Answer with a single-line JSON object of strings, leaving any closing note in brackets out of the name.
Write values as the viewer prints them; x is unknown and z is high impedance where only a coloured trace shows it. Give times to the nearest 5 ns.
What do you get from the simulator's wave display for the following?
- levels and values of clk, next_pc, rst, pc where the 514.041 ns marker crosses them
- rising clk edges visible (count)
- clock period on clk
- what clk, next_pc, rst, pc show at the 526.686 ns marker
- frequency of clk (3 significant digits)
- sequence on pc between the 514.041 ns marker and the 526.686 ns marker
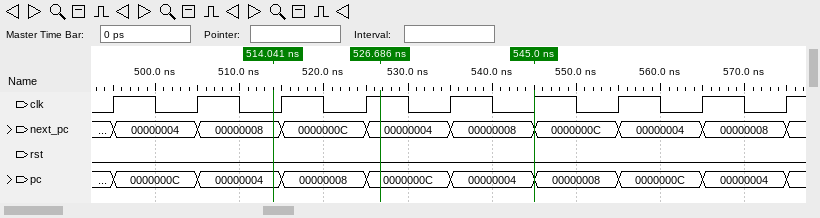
{"levels and values of clk, next_pc, rst, pc where the 514.041 ns marker crosses them": "clk=0, next_pc=00000008, rst=0, pc=00000004", "rising clk edges visible": "9", "clock period on clk": "10 ns", "what clk, next_pc, rst, pc show at the 526.686 ns marker": "clk=1, next_pc=00000004, rst=0, pc=0000000C", "frequency of clk": "100 MHz", "sequence on pc between the 514.041 ns marker and the 526.686 ns marker": "00000004, 00000008, 0000000C"}
